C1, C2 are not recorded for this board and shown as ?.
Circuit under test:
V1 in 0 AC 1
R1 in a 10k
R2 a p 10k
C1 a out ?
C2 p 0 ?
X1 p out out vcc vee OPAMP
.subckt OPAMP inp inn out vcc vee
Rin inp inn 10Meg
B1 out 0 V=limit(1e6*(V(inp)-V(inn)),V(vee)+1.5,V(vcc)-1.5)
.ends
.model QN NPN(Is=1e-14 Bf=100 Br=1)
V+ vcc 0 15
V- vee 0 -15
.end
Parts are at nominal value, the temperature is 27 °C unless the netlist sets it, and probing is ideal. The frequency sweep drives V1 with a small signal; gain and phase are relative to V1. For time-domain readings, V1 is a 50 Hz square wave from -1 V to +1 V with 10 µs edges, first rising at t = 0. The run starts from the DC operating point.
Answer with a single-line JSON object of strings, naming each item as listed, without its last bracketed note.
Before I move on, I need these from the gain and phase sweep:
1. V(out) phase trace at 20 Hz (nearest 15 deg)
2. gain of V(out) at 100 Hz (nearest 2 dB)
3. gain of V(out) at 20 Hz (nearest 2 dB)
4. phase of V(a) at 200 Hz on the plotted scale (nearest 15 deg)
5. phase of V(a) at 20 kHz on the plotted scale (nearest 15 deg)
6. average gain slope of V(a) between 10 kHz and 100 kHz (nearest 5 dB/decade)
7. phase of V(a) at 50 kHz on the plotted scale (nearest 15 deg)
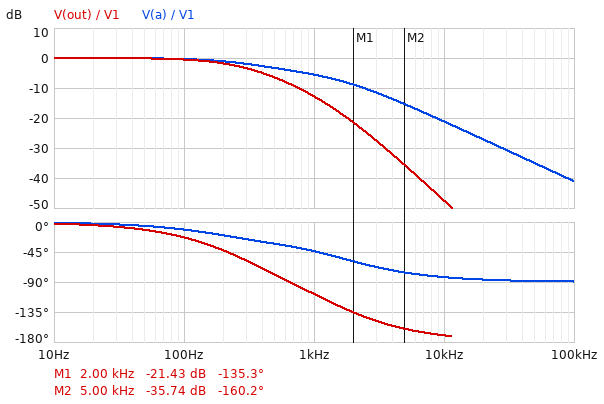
{"V(out) phase trace at 20 Hz": "0 deg", "gain of V(out) at 100 Hz": "0 dB", "gain of V(out) at 20 Hz": "0 dB", "phase of V(a) at 200 Hz on the plotted scale": "-15 deg", "phase of V(a) at 20 kHz on the plotted scale": "-90 deg", "average gain slope of V(a) between 10 kHz and 100 kHz": "-20 dB/decade", "phase of V(a) at 50 kHz on the plotted scale": "-90 deg"}
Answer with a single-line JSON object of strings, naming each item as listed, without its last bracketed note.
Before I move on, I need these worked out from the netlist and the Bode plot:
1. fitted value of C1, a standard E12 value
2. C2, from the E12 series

{"fitted value of C1, a standard E12 value": "18 nF", "C2, from the E12 series": "33 nF"}
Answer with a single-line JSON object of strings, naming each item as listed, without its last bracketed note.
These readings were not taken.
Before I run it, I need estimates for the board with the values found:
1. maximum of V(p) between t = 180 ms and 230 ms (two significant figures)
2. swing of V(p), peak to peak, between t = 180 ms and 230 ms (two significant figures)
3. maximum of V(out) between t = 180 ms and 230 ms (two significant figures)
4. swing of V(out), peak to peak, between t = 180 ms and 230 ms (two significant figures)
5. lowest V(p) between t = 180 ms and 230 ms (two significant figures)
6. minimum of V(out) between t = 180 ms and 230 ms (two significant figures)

{"maximum of V(p) between t = 180 ms and 230 ms": "1.0 V", "swing of V(p), peak to peak, between t = 180 ms and 230 ms": "2.0 V", "maximum of V(out) between t = 180 ms and 230 ms": "1.0 V", "swing of V(out), peak to peak, between t = 180 ms and 230 ms": "2.0 V", "lowest V(p) between t = 180 ms and 230 ms": "-1.0 V", "minimum of V(out) between t = 180 ms and 230 ms": "-1.0 V"}
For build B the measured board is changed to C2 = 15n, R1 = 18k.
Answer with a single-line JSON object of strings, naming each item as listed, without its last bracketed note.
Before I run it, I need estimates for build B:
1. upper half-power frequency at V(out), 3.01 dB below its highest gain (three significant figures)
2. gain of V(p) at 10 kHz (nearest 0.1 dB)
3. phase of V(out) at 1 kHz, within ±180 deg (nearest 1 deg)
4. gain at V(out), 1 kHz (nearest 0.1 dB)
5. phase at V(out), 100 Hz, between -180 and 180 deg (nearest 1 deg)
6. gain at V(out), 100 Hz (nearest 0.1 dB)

{"upper half-power frequency at V(out), 3.01 dB below its highest gain": "498 Hz", "gain of V(p) at 10 kHz": "-45.7 dB", "phase of V(out) at 1 kHz, within ±180 deg": "-109 deg", "gain at V(out), 1 kHz": "-8.9 dB", "phase at V(out), 100 Hz, between -180 and 180 deg": "-15 deg", "gain at V(out), 100 Hz": "-0.1 dB"}
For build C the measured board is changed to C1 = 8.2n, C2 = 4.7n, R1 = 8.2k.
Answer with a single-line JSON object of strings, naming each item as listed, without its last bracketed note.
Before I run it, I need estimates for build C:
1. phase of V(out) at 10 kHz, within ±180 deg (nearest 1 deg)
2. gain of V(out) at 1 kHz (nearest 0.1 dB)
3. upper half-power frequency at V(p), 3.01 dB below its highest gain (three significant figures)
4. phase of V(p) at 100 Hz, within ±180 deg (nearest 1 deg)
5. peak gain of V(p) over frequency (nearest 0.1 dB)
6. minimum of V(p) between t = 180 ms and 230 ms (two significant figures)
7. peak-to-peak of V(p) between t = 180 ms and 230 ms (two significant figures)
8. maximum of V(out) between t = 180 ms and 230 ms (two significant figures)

{"phase of V(out) at 10 kHz, within ±180 deg": "-155 deg", "gain of V(out) at 1 kHz": "-0.2 dB", "upper half-power frequency at V(p), 3.01 dB below its highest gain": "2.62 kHz", "phase of V(p) at 100 Hz, within ±180 deg": "-3 deg", "peak gain of V(p) over frequency": "0 dB", "minimum of V(p) between t = 180 ms and 230 ms": "-1.1 V", "peak-to-peak of V(p) between t = 180 ms and 230 ms": "2.1 V", "maximum of V(out) between t = 180 ms and 230 ms": "1.1 V"}
